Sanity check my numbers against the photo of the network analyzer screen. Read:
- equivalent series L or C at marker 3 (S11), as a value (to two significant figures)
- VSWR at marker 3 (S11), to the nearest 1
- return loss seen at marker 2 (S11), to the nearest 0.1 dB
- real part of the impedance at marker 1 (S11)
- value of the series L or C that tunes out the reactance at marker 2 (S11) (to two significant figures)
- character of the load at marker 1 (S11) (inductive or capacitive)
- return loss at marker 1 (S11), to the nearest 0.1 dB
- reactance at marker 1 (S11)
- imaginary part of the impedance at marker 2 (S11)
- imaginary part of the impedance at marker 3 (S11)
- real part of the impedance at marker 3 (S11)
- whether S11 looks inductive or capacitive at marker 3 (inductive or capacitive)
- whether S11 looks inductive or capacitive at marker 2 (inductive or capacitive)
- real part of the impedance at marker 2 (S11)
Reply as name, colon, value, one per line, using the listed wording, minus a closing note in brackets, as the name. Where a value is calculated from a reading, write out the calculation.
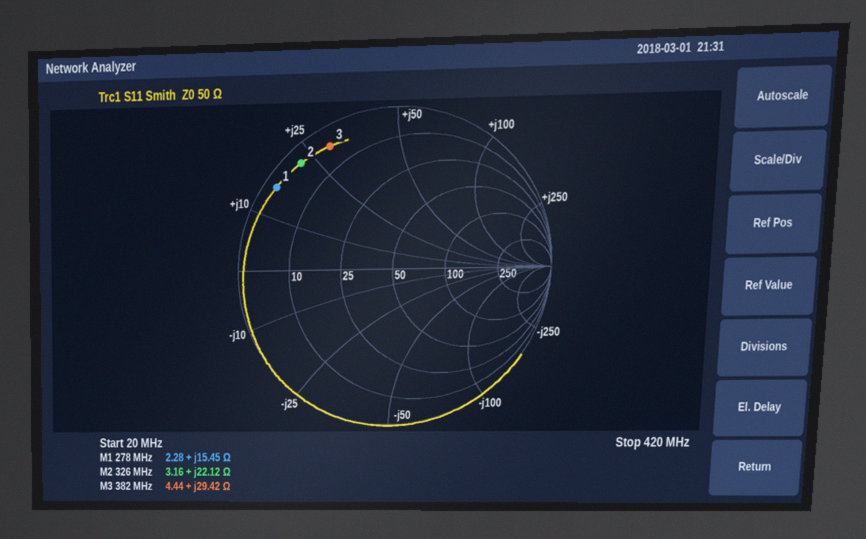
equivalent series L or C at marker 3 (S11), as a value: L = 29.42 Ω/(2π × 382 MHz) ≈ 12 nH
VSWR at marker 3 (S11), to the nearest 1: 15
return loss seen at marker 2 (S11), to the nearest 0.1 dB: 0.9 dB
real part of the impedance at marker 1: 2.28 Ω
value of the series L or C that tunes out the reactance at marker 2 (S11): C = 1/(2π × 326 MHz × 22.12 Ω) ≈ 22 pF
character of the load at marker 1 (S11): inductive
return loss at marker 1 (S11), to the nearest 0.1 dB: 0.7 dB
reactance at marker 1: +15.45 Ω
imaginary part of the impedance at marker 2: +22.12 Ω
imaginary part of the impedance at marker 3: +29.42 Ω
real part of the impedance at marker 3: 4.44 Ω
whether S11 looks inductive or capacitive at marker 3: inductive
whether S11 looks inductive or capacitive at marker 2: inductive
real part of the impedance at marker 2: 3.16 Ω
